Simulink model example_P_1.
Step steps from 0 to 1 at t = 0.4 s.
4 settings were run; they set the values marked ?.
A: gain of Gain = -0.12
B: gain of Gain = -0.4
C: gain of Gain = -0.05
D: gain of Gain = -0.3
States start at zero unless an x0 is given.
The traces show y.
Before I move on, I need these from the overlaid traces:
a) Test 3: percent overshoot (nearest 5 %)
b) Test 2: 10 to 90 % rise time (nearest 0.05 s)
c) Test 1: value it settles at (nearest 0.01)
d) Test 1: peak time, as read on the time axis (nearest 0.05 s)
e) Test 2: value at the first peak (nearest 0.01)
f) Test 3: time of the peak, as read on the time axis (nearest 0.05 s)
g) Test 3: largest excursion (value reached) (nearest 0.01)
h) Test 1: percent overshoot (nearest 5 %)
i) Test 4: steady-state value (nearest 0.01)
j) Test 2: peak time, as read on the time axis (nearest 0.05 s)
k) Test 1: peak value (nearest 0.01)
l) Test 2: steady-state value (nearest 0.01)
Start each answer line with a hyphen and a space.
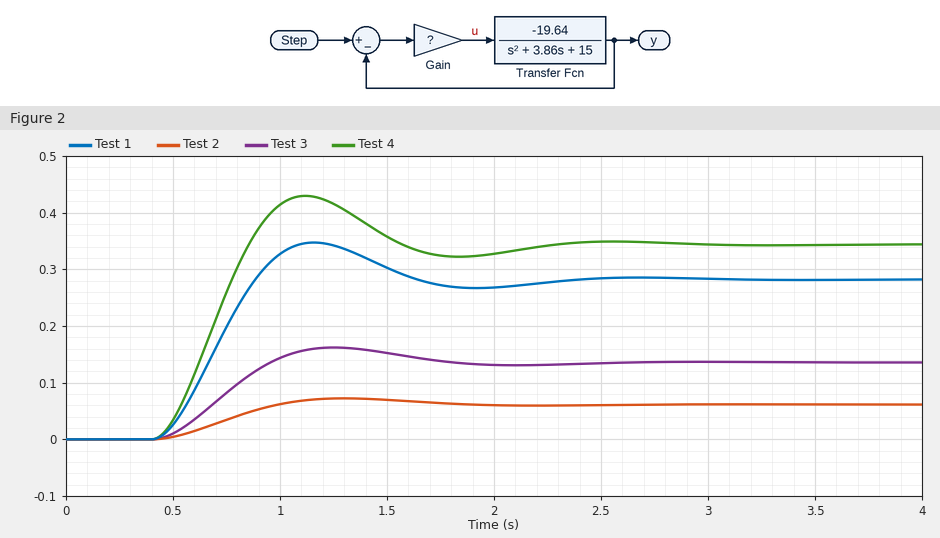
- 20 %
- 0.40 s
- 0.28
- 1.15 s
- 0.07
- 1.25 s
- 0.16
- 25 %
- 0.34
- 1.30 s
- 0.35
- 0.06
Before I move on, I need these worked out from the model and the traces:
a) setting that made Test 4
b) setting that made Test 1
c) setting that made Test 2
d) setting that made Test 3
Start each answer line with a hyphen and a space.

- B
- D
- C
- A
